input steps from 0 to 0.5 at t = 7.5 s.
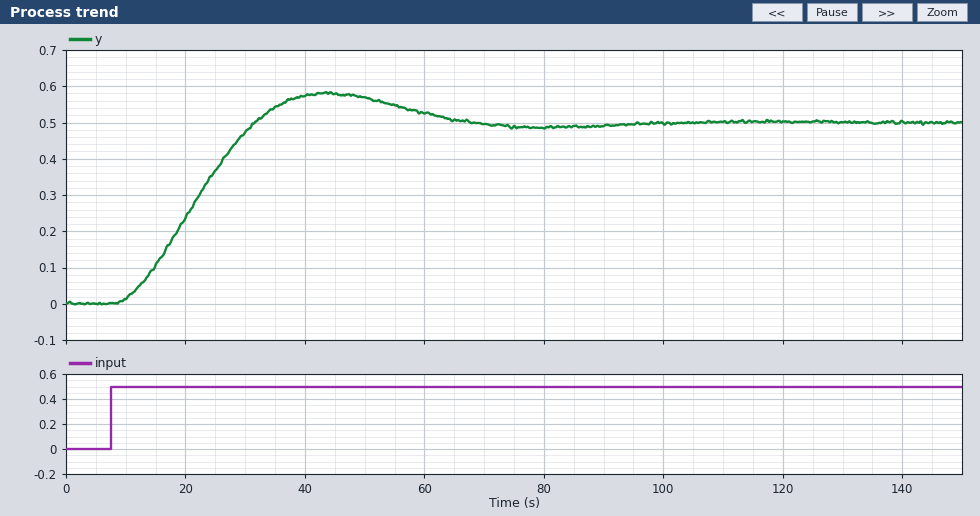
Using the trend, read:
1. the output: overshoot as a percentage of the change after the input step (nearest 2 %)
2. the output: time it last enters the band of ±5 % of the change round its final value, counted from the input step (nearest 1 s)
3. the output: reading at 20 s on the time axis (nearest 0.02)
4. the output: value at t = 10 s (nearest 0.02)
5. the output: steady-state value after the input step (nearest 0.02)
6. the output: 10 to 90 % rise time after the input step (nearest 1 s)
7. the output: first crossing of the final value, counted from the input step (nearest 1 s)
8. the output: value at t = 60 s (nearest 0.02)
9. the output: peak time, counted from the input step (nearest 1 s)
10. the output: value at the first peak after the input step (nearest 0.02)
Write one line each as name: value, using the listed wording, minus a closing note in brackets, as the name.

the output: overshoot as a percentage of the change after the input step: 16 %
the output: time it last enters the band of ±5 % of the change round its final value, counted from the input step: 53 s
the output: reading at 20 s on the time axis: 0.24
the output: value at t = 10 s: 0.02
the output: steady-state value after the input step: 0.50
the output: 10 to 90 % rise time after the input step: 16 s
the output: first crossing of the final value, counted from the input step: 24 s
the output: value at t = 60 s: 0.52
the output: peak time, counted from the input step: 36 s
the output: value at the first peak after the input step: 0.58
